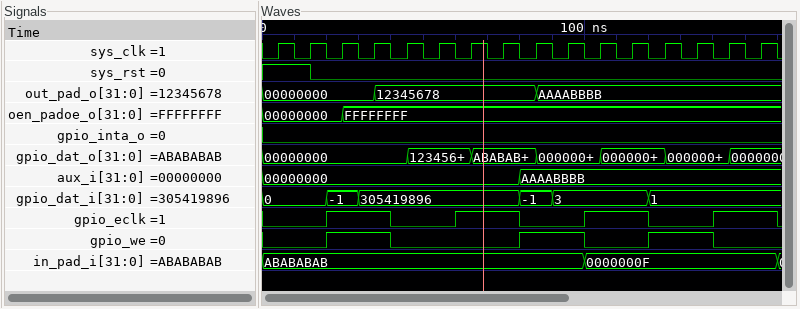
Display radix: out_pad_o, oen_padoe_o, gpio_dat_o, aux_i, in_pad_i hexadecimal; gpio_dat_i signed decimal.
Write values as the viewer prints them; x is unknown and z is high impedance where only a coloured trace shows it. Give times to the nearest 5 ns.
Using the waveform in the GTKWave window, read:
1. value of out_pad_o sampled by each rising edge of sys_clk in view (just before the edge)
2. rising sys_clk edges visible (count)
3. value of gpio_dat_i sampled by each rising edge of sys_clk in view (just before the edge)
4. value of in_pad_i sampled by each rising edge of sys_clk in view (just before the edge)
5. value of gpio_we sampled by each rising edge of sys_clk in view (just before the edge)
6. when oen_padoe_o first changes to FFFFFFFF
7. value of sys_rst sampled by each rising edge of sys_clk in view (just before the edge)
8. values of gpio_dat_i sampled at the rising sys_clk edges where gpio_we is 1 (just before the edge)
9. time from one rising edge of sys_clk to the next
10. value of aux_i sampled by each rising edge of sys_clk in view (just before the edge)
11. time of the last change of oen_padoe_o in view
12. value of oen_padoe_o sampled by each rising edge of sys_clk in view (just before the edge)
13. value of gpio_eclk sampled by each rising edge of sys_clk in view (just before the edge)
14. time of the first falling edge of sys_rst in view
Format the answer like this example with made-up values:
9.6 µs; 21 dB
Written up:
00000000, 00000000, 00000000, 00000000, 12345678, 12345678, 12345678, 12345678, 12345678, AAAABBBB, AAAABBBB, AAAABBBB, AAAABBBB, AAAABBBB, AAAABBBB, AAAABBBB; 16; 0, 0, -1, 305419896, 305419896, 305419896, 305419896, 305419896, -1, 3, 3, 3, 1, 1, 1, 1; ABABABAB, ABABABAB, ABABABAB, ABABABAB, ABABABAB, ABABABAB, ABABABAB, ABABABAB, ABABABAB, ABABABAB, 0000000F, 0000000F, 0000000F, 0000000F, 0000000F, 0000000F; 0 0 1 1 0 0 0 0 1 1 0 0 1 1 0 0; 25 ns; 1 1 0 0 0 0 0 0 0 0 0 0 0 0 0 0; -1, 305419896, -1, 3, 1, 1; 10 ns; 00000000, 00000000, 00000000, 00000000, 00000000, 00000000, 00000000, 00000000, AAAABBBB, AAAABBBB, AAAABBBB, AAAABBBB, AAAABBBB, AAAABBBB, AAAABBBB, AAAABBBB; 25 ns; 00000000, 00000000, 00000000, FFFFFFFF, FFFFFFFF, FFFFFFFF, FFFFFFFF, FFFFFFFF, FFFFFFFF, FFFFFFFF, FFFFFFFF, FFFFFFFF, FFFFFFFF, FFFFFFFF, FFFFFFFF, FFFFFFFF; 0 0 1 1 0 0 1 1 0 0 1 1 0 0 1 1; 15 ns
